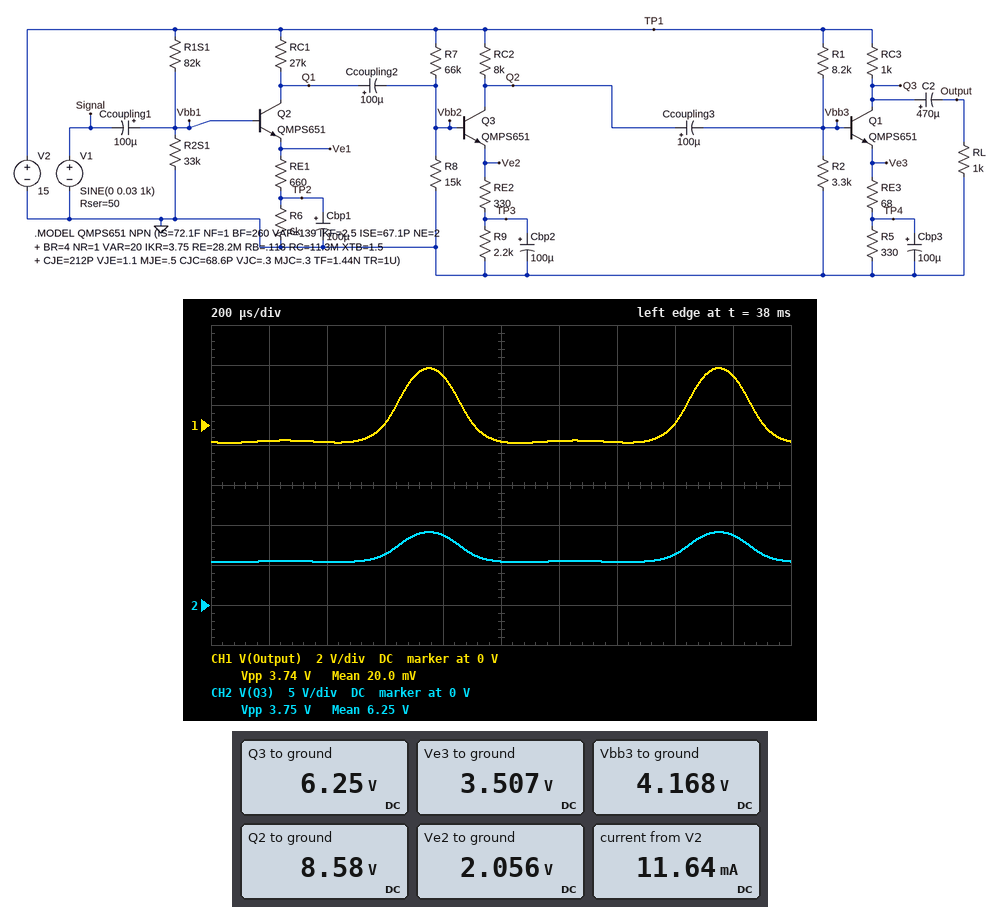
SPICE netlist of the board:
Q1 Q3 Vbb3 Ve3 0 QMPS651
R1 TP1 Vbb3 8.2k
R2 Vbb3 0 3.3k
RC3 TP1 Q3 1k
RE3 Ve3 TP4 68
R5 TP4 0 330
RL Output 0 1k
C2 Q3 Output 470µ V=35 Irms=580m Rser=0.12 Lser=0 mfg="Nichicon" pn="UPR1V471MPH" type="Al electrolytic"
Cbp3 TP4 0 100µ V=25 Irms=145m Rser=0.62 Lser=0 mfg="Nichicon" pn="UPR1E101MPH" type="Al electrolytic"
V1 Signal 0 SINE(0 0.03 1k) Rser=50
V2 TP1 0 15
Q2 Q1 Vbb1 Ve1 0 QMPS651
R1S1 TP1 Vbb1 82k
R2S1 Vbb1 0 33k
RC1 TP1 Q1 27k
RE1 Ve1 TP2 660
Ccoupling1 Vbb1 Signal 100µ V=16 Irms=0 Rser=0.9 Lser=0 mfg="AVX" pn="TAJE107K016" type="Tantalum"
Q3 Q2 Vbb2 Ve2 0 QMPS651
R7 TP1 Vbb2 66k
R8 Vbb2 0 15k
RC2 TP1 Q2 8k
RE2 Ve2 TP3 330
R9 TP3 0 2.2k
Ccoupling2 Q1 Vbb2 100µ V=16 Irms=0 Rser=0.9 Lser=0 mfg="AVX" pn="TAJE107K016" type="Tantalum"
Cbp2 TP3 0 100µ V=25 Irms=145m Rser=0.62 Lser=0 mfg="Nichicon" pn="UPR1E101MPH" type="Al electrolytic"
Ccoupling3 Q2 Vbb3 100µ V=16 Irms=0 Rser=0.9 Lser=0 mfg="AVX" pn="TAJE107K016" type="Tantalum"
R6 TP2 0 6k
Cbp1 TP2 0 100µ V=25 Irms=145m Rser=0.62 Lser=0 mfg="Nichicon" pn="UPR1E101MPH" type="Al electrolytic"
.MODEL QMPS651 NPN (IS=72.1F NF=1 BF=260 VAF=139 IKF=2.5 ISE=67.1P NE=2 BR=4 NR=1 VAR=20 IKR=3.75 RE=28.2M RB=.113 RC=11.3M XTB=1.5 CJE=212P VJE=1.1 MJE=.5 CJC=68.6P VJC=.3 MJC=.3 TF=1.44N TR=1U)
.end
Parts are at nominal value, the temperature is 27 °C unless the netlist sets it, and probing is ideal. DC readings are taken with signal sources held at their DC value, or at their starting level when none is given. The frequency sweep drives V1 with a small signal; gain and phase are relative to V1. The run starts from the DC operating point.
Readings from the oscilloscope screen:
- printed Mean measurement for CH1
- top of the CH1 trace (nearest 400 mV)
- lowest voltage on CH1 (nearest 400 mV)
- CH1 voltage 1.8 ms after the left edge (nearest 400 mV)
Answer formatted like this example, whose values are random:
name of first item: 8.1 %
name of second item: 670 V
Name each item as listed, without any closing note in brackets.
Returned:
printed Mean measurement for CH1: 20.0 mV
top of the CH1 trace: 2.8 V
lowest voltage on CH1: -800 mV
CH1 voltage 1.8 ms after the left edge: 2.4 V
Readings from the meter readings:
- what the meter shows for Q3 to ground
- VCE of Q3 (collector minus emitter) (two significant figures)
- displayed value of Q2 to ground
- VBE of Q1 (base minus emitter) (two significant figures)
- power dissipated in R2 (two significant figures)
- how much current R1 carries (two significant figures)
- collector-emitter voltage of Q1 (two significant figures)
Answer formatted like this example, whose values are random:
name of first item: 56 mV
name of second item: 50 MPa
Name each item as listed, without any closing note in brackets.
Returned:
what the meter shows for Q3 to ground: 6.25 V
VCE of Q3 (collector minus emitter): 6.5 V
displayed value of Q2 to ground: 8.58 V
VBE of Q1 (base minus emitter): 660 mV
power dissipated in R2: 5.3 mW
how much current R1 carries: 1.3 mA
collector-emitter voltage of Q1: 2.7 V
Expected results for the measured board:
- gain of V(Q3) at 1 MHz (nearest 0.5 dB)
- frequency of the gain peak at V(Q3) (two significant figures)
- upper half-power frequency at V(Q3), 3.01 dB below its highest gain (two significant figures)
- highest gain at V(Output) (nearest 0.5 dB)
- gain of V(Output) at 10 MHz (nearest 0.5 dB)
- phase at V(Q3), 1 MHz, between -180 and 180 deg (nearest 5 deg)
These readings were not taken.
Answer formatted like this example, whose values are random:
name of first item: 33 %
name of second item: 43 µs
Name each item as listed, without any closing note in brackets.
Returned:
gain of V(Q3) at 1 MHz: 17.0 dB
frequency of the gain peak at V(Q3): 110 kHz
upper half-power frequency at V(Q3), 3.01 dB below its highest gain: 360 kHz
highest gain at V(Output): 27.0 dB
gain of V(Output) at 10 MHz: -0.5 dB
phase at V(Q3), 1 MHz, between -180 and 180 deg: -80 deg
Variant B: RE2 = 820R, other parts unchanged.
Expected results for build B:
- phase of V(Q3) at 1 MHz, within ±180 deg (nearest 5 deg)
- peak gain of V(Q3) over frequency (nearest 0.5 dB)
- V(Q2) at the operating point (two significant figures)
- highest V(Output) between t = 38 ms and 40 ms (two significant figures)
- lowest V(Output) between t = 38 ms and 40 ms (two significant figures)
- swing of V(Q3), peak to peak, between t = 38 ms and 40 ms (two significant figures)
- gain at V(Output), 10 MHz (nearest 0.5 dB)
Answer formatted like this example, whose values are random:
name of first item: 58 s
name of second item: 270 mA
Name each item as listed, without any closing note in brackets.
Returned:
phase of V(Q3) at 1 MHz, within ±180 deg: -85 deg
peak gain of V(Q3) over frequency: 20.0 dB
V(Q2) at the operating point: 9.6 V
highest V(Output) between t = 38 ms and 40 ms: 1.3 V
lowest V(Output) between t = 38 ms and 40 ms: -380 mV
swing of V(Q3), peak to peak, between t = 38 ms and 40 ms: 1.7 V
gain at V(Output), 10 MHz: -4.0 dB
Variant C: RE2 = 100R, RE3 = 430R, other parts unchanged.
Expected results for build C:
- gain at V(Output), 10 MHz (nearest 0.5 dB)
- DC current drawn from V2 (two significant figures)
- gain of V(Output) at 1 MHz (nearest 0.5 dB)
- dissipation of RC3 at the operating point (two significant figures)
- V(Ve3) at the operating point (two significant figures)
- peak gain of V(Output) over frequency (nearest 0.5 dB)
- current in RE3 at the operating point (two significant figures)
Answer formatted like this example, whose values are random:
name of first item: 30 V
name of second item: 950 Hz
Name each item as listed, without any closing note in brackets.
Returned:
gain at V(Output), 10 MHz: 2.5 dB
DC current drawn from V2: 7.6 mA
gain of V(Output) at 1 MHz: 18.5 dB
dissipation of RC3 at the operating point: 22 mW
V(Ve3) at the operating point: 3.6 V
peak gain of V(Output) over frequency: 21.5 dB
current in RE3 at the operating point: 4.7 mA
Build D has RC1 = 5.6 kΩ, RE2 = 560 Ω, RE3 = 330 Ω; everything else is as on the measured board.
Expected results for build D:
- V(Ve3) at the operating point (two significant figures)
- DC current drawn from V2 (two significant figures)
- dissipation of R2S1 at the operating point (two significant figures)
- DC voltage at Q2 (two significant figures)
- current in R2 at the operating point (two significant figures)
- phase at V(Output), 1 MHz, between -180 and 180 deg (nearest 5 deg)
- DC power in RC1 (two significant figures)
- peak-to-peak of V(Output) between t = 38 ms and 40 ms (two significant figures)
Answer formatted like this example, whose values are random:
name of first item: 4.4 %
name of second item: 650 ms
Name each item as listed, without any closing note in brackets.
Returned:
V(Ve3) at the operating point: 3.6 V
DC current drawn from V2: 8.3 mA
dissipation of R2S1 at the operating point: 520 µW
DC voltage at Q2: 9.1 V
current in R2 at the operating point: 1.3 mA
phase at V(Output), 1 MHz, between -180 and 180 deg: 50 deg
DC power in RC1: 1.5 mW
peak-to-peak of V(Output) between t = 38 ms and 40 ms: 1.3 V
